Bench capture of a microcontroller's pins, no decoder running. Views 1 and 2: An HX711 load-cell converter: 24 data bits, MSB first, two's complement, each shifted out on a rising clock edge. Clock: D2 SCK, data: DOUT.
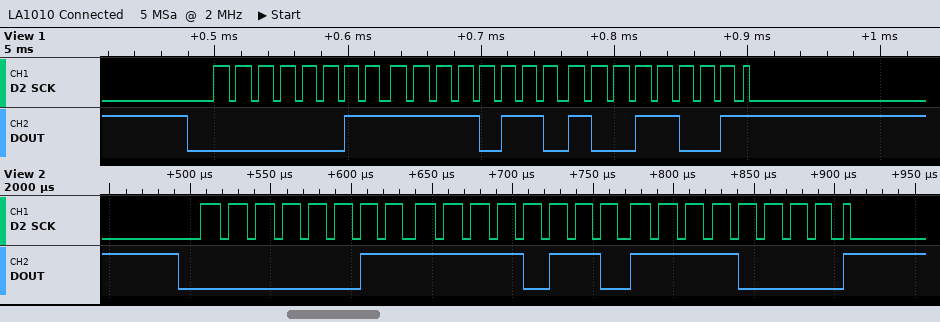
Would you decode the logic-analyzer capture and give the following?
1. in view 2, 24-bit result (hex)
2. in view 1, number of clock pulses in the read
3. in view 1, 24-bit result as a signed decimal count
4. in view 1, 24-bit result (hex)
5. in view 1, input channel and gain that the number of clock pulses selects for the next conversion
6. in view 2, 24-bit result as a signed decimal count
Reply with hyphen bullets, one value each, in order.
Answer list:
- 0x03F6F0
- 25
- 259737
- 0x03F699
- channel A, gain 128
- 259824
